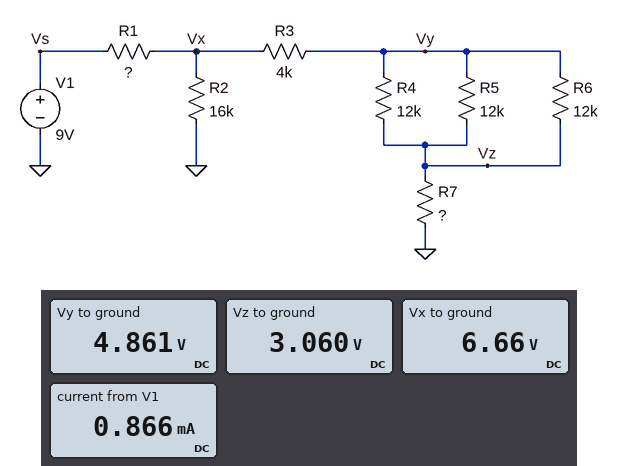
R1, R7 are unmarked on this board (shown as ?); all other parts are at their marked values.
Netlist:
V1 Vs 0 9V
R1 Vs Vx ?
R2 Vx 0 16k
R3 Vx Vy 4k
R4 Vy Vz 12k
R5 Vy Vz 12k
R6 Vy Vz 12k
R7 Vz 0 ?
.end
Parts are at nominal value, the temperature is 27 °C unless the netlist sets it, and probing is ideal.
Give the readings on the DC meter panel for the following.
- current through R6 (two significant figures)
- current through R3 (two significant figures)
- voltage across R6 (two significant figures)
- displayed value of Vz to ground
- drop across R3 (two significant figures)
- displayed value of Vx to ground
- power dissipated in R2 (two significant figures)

150 µA
450 µA
1.8 V
3.060 V
1.8 V
6.66 V
2.8 mW
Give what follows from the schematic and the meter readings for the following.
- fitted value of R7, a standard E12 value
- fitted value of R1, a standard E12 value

6.8 kΩ
2.7 kΩ
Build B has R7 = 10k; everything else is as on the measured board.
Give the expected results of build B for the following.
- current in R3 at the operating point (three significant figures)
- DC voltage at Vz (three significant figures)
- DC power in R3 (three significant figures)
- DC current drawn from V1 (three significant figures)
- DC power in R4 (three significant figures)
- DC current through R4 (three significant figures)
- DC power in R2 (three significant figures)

379 µA
3.79 V
575 µW
806 µA
192 µW
126 µA
2.91 mW
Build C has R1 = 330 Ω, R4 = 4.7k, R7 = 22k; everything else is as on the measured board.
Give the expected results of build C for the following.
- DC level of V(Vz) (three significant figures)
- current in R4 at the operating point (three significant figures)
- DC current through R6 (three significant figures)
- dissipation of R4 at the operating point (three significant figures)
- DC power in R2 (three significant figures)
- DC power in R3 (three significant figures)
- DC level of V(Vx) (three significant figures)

6.70 V
171 µA
66.9 µA
137 µW
4.75 mW
371 µW
8.72 V
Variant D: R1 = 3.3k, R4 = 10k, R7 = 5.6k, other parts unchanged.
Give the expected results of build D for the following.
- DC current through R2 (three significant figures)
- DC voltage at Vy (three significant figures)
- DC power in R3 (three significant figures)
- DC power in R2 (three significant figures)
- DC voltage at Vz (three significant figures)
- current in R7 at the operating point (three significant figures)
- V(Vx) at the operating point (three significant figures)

387 µA
4.34 V
861 µW
2.40 mW
2.60 V
464 µA
6.19 V
